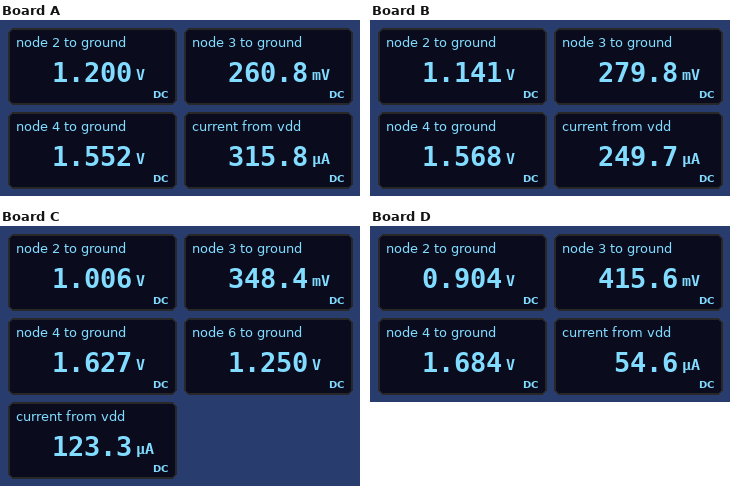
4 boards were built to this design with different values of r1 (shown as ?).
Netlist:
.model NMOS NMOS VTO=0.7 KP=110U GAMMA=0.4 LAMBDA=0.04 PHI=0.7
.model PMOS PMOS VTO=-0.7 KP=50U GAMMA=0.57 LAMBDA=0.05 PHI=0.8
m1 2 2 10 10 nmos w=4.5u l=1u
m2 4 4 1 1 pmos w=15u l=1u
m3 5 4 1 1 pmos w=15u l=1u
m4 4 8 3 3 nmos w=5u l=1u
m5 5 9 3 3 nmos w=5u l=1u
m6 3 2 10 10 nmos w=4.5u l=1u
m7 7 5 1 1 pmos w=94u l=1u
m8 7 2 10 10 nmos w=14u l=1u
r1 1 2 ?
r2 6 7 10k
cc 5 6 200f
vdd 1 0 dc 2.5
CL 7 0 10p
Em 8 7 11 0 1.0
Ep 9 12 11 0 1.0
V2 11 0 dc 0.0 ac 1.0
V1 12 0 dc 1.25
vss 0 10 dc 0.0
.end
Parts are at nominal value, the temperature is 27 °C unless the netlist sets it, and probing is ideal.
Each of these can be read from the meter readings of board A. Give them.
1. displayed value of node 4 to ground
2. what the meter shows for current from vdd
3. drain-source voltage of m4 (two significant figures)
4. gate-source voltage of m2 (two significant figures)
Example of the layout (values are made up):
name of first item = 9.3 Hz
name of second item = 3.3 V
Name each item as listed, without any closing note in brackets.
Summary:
displayed value of node 4 to ground = 1.552 V
what the meter shows for current from vdd = 315.8 µA
drain-source voltage of m4 = 1.3 V
gate-source voltage of m2 = -950 mV
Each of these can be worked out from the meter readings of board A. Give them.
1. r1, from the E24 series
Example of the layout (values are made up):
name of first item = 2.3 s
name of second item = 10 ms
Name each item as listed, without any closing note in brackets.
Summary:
r1, from the E24 series = 20 kΩ
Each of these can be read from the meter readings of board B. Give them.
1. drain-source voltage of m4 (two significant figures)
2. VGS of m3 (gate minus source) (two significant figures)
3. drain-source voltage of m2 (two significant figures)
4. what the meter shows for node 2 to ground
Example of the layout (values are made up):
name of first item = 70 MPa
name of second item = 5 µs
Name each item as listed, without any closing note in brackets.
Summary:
drain-source voltage of m4 = 1.3 V
VGS of m3 (gate minus source) = -930 mV
drain-source voltage of m2 = -930 mV
what the meter shows for node 2 to ground = 1.141 V
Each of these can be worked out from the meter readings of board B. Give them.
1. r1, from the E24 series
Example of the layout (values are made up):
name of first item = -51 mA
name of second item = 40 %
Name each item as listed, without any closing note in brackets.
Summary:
r1, from the E24 series = 27 kΩ
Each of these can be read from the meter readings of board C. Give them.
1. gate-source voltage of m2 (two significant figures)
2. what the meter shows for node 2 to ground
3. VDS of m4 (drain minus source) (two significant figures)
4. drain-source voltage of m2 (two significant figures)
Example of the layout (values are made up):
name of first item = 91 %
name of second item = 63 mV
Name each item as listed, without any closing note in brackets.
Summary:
gate-source voltage of m2 = -870 mV
what the meter shows for node 2 to ground = 1.006 V
VDS of m4 (drain minus source) = 1.3 V
drain-source voltage of m2 = -870 mV
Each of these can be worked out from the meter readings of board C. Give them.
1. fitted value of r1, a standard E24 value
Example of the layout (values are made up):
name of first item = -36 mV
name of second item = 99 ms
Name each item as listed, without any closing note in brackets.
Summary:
fitted value of r1, a standard E24 value = 62 kΩ
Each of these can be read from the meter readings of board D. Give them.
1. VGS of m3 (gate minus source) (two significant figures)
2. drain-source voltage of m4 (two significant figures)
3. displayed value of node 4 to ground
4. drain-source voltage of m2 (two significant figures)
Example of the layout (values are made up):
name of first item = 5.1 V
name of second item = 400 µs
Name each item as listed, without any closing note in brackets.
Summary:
VGS of m3 (gate minus source) = -820 mV
drain-source voltage of m4 = 1.3 V
displayed value of node 4 to ground = 1.684 V
drain-source voltage of m2 = -820 mV
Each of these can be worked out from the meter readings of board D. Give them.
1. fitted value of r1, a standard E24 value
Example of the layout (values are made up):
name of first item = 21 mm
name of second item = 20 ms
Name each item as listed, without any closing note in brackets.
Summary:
fitted value of r1, a standard E24 value = 150 kΩ
